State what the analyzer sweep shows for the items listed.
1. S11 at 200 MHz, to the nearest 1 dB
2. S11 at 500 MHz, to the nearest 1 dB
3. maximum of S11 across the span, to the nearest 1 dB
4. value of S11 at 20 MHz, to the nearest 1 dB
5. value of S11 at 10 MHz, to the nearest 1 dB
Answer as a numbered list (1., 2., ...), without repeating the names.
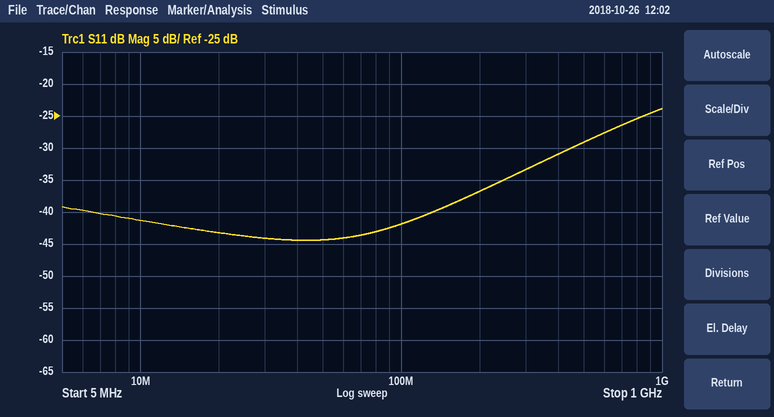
1. -37 dB
2. -29 dB
3. -24 dB
4. -43 dB
5. -41 dB
